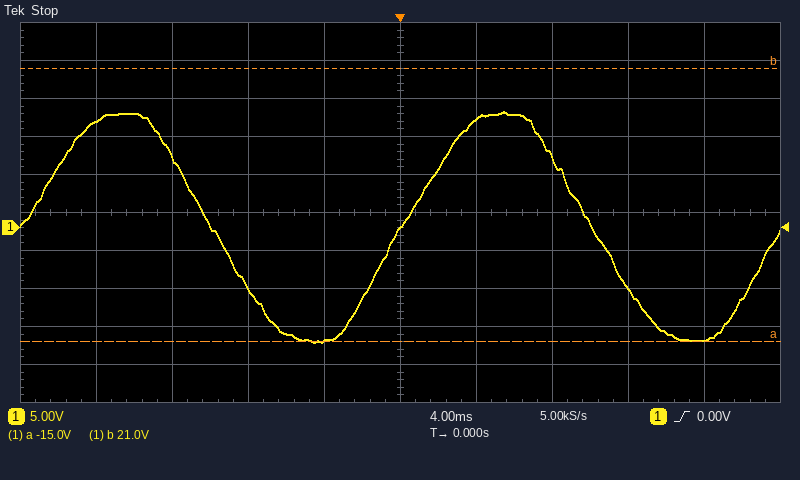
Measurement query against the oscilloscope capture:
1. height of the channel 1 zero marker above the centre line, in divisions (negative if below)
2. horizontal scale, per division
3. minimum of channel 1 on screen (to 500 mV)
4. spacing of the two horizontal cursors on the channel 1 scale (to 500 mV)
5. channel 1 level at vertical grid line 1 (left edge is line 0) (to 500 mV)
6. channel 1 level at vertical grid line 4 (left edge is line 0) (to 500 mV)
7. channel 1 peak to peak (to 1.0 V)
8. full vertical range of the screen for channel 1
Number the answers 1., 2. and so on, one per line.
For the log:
1. -0.4 div
2. 4 ms
3. -15.0 V
4. 36.0 V
5. 14.0 V
6. -15.0 V
7. 30.0 V
8. 50 V
